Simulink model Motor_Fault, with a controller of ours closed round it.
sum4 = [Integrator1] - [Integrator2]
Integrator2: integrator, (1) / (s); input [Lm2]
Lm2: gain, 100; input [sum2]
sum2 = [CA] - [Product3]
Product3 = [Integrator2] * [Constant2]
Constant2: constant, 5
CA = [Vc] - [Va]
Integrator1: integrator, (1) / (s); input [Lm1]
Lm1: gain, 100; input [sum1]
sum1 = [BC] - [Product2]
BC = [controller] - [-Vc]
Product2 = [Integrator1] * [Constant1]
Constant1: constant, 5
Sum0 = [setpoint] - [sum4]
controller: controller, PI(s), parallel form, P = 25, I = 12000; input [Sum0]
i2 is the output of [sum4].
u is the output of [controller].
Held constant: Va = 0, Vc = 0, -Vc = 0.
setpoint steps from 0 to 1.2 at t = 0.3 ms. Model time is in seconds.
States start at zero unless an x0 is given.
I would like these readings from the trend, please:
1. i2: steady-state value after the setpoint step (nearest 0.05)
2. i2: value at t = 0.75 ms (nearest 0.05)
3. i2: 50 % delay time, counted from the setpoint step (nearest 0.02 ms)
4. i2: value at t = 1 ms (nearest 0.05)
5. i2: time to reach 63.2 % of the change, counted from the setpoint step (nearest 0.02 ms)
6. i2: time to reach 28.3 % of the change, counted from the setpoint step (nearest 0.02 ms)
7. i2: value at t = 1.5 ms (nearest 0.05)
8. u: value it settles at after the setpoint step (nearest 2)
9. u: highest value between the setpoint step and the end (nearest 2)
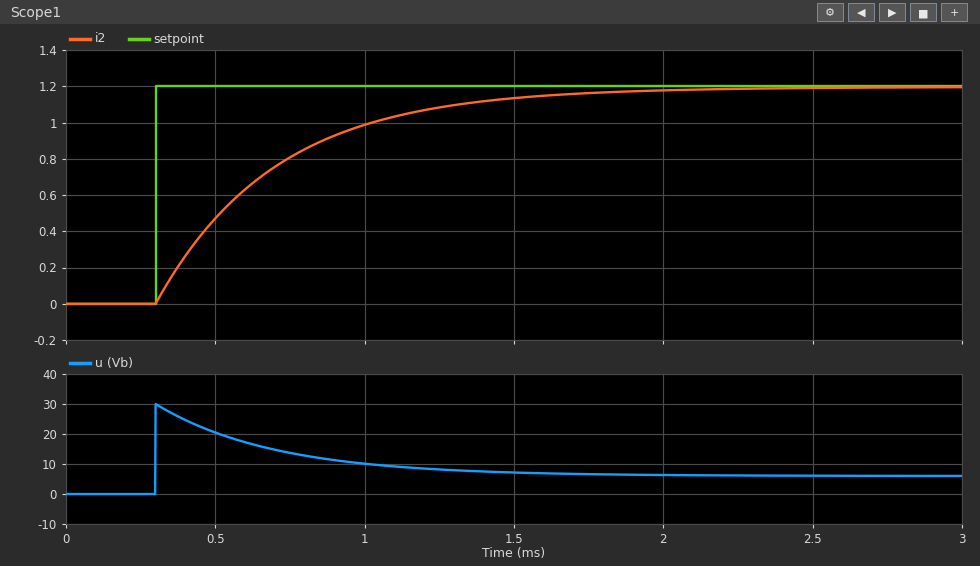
1.20
0.80
0.28 ms
1.00
0.40 ms
0.14 ms
1.15
6
30
